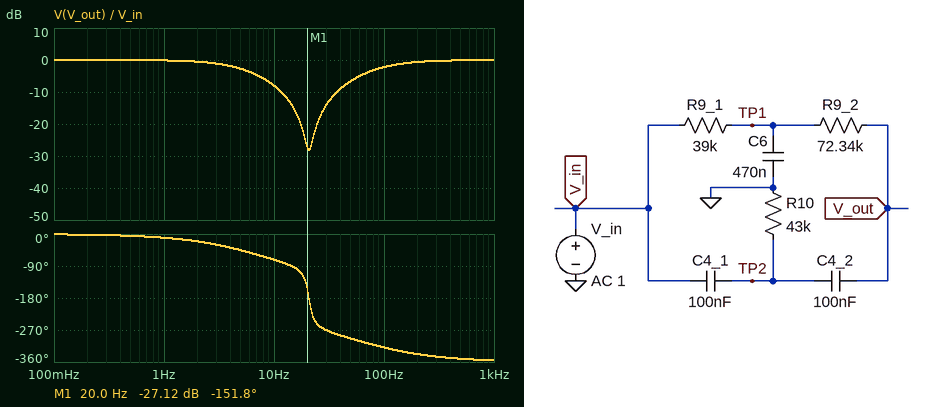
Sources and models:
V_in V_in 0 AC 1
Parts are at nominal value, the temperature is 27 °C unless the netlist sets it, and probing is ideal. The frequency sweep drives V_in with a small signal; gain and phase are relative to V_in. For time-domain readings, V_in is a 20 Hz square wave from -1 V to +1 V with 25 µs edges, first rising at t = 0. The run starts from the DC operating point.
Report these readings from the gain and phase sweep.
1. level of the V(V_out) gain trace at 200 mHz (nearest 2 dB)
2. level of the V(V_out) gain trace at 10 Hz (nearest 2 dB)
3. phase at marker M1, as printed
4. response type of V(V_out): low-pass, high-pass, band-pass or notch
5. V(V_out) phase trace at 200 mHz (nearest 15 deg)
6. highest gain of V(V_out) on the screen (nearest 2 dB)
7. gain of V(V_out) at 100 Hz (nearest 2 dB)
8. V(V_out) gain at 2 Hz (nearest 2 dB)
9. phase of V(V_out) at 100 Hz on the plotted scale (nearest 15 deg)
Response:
0 dB
-8 dB
-151.8 deg
notch
0 deg
0 dB
-2 dB
0 dB
-315 deg
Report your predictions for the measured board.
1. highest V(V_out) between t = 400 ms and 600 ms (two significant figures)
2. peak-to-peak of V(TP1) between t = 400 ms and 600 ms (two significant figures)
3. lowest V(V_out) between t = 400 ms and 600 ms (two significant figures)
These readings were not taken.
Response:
1.7 V
1.1 V
-1.7 V
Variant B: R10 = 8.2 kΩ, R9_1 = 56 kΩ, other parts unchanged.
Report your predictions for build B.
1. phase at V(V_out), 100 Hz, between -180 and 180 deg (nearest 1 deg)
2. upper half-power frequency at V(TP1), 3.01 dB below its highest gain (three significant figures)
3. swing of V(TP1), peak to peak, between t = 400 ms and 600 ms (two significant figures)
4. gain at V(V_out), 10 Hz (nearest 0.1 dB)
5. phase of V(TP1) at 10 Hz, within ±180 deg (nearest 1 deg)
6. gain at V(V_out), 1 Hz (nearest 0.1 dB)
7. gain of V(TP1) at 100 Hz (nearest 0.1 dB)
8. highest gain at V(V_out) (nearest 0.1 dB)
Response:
77 deg
4.79 Hz
780 mV
-8.4 dB
-59 deg
-0.2 dB
-23.5 dB
0 dB
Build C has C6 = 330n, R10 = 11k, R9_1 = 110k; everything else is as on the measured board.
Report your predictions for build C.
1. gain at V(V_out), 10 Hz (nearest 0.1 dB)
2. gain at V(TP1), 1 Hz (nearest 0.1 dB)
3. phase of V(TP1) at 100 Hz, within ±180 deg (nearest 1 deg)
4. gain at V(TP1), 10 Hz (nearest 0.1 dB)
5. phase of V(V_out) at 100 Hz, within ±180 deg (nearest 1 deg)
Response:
-11.6 dB
-0.4 dB
-55 deg
-10.1 dB
70 deg
